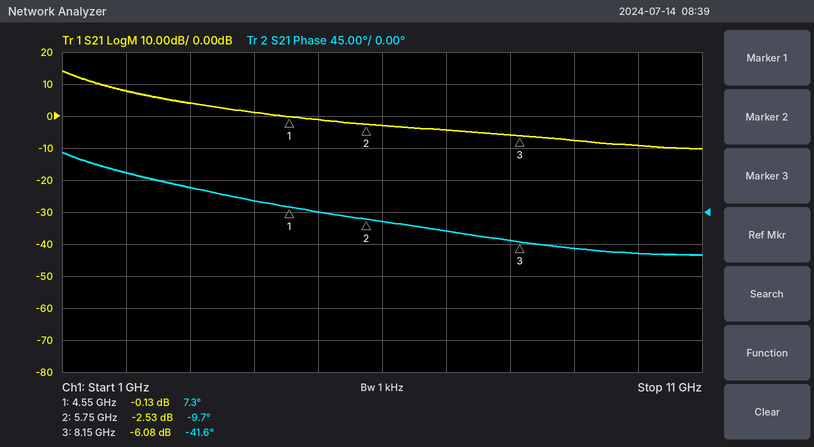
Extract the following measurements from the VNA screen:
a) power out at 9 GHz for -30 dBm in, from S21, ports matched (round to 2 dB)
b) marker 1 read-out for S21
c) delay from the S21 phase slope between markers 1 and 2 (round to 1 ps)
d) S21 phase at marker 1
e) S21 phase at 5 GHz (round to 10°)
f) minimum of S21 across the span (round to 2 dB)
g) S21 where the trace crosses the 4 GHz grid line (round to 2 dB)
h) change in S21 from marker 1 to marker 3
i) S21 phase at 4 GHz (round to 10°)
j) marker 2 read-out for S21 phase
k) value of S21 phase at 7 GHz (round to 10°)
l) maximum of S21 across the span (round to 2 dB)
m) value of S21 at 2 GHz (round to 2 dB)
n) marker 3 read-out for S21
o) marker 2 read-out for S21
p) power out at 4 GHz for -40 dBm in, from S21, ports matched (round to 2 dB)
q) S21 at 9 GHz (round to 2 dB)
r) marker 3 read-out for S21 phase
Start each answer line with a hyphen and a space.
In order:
- -38 dBm
- -0.13 dB
- 39 ps
- 7.3°
- 0°
- -10 dB
- 2 dB
- -5.95 dB
- 20°
- -9.7°
- -30°
- 14 dB
- 8 dB
- -6.08 dB
- -2.53 dB
- -38 dBm
- -8 dB
- -41.6°
